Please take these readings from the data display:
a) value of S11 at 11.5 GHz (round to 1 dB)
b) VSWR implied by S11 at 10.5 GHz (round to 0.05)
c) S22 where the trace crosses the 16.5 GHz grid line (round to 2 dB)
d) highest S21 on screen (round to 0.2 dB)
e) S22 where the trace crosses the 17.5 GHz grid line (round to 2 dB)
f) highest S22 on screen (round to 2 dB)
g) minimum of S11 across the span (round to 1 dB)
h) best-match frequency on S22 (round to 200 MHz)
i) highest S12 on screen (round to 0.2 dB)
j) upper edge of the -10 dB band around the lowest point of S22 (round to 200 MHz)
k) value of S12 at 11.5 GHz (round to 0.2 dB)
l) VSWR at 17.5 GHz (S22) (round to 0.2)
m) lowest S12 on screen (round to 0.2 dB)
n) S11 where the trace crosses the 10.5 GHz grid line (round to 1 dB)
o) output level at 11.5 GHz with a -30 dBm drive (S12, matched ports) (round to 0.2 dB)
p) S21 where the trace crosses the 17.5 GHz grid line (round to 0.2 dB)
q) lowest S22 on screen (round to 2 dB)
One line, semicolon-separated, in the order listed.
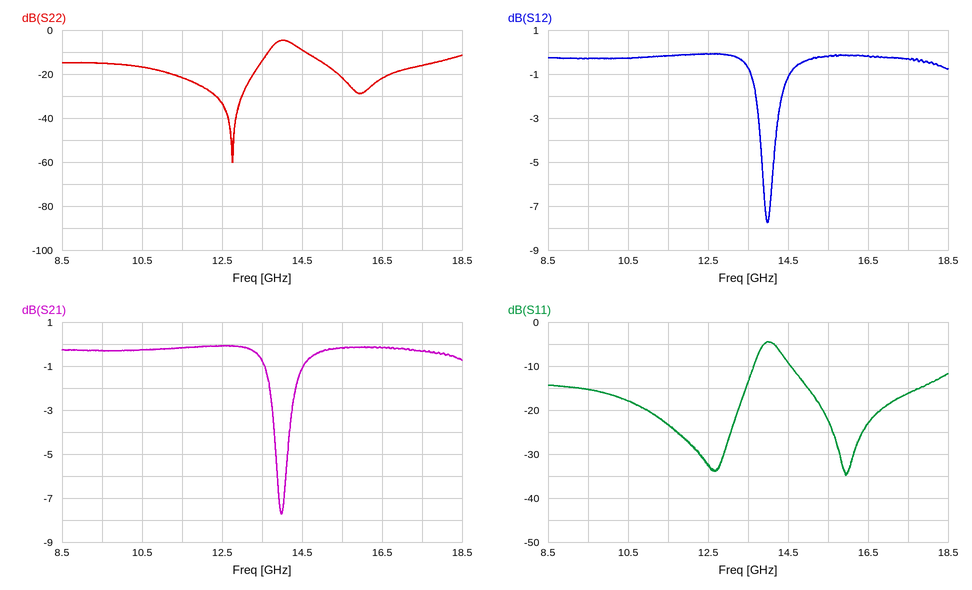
-23 dB; 1.30; -22 dB; 0.0 dB; -16 dB; -4 dB; -35 dB; 12.8 GHz; 0.0 dB; 13.6 GHz; -0.2 dB; 1.4; -7.8 dB; -18 dB; -30.2 dBm; -0.4 dB; -60 dB
